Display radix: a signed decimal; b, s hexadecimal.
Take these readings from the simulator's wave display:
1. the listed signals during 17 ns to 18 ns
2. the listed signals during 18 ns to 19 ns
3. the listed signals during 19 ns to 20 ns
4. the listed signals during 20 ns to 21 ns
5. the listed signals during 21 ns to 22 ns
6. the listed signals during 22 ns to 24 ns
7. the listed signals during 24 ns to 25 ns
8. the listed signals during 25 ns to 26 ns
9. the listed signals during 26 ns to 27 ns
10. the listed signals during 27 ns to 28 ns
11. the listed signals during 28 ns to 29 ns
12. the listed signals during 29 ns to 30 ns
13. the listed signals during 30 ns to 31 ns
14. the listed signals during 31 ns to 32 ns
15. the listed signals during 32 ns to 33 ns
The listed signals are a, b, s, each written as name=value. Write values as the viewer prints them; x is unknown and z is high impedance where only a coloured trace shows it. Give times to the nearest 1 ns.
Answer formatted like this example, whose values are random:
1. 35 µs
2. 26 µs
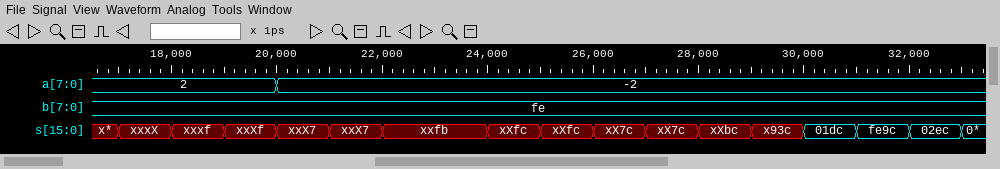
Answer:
1. a=2, b=fe, s=xxxX
2. a=2, b=fe, s=xxxf
3. a=2, b=fe, s=xxXf
4. a=-2, b=fe, s=xxX7
5. a=-2, b=fe, s=xxX7
6. a=-2, b=fe, s=xxfb
7. a=-2, b=fe, s=xXfc
8. a=-2, b=fe, s=xXfc
9. a=-2, b=fe, s=xX7c
10. a=-2, b=fe, s=xX7c
11. a=-2, b=fe, s=xXbc
12. a=-2, b=fe, s=x93c
13. a=-2, b=fe, s=01dc
14. a=-2, b=fe, s=fe9c
15. a=-2, b=fe, s=02ec
